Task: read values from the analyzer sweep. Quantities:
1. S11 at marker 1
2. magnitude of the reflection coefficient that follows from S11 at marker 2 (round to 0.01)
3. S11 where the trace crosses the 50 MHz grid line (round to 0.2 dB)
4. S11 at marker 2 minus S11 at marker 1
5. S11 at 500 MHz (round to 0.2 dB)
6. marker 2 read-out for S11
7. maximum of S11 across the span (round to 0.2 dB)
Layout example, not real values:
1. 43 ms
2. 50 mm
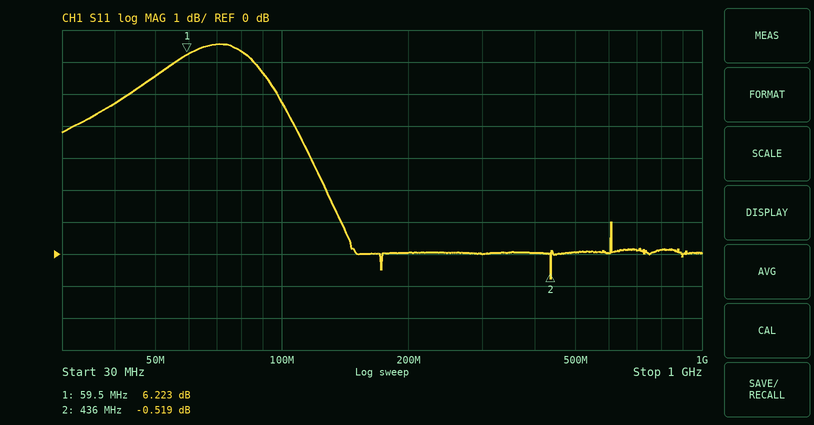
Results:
1. 6.223 dB
2. 0.94
3. 5.6 dB
4. -6.742 dB
5. 0.0 dB
6. -0.519 dB
7. 6.6 dB
